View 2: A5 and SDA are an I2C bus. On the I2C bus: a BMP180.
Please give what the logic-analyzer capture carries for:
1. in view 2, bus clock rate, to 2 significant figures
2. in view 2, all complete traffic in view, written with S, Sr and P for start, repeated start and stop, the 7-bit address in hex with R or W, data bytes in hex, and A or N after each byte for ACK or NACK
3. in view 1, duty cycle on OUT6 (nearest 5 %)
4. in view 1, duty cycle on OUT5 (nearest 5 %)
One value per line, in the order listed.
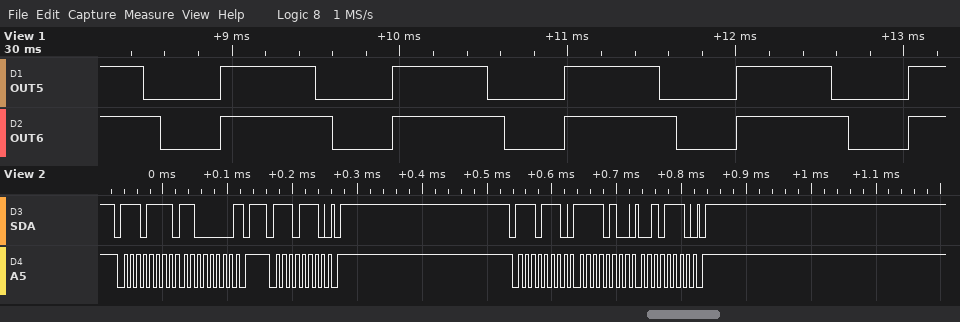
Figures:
100 kHz
S 77R A C0 N P S 77W A P S 77W A F4 A 2E A P
65 %
55 %
